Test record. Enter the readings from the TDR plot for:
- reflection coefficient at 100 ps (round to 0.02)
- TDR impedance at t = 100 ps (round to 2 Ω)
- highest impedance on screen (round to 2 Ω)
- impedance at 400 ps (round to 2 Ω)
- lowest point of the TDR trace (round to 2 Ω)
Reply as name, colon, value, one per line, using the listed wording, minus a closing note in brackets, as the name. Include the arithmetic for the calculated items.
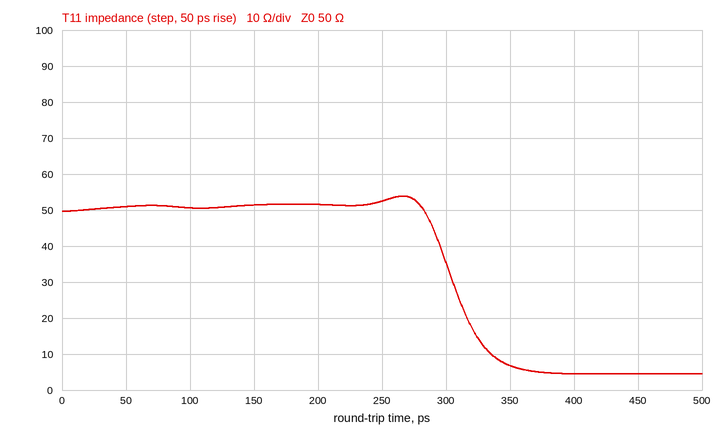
reflection coefficient at 100 ps: (50 − 50)/(50 + 50) ≈ 0.00
TDR impedance at t = 100 ps: 50 Ω
highest impedance on screen: 54 Ω
impedance at 400 ps: 4 Ω
lowest point of the TDR trace: 4 Ω
